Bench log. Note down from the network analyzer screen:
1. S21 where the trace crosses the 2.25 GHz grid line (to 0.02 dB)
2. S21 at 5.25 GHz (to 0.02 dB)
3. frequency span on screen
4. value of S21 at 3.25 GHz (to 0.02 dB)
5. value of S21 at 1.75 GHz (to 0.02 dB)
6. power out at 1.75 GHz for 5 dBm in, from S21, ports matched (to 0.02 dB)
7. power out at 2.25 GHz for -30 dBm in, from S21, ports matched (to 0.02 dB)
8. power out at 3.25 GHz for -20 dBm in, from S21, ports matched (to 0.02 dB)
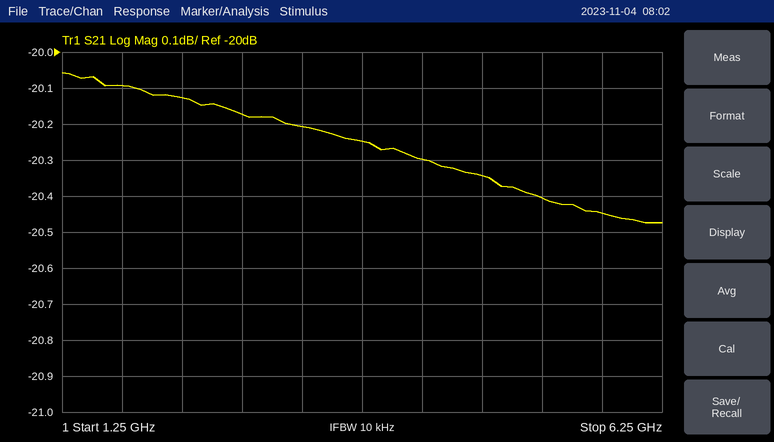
-20.12 dB
-20.40 dB
5 GHz
-20.20 dB
-20.10 dB
-15.10 dBm
-50.12 dBm
-40.20 dBm
